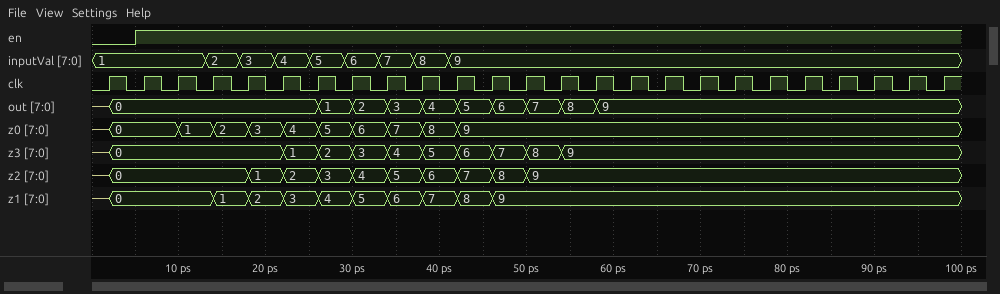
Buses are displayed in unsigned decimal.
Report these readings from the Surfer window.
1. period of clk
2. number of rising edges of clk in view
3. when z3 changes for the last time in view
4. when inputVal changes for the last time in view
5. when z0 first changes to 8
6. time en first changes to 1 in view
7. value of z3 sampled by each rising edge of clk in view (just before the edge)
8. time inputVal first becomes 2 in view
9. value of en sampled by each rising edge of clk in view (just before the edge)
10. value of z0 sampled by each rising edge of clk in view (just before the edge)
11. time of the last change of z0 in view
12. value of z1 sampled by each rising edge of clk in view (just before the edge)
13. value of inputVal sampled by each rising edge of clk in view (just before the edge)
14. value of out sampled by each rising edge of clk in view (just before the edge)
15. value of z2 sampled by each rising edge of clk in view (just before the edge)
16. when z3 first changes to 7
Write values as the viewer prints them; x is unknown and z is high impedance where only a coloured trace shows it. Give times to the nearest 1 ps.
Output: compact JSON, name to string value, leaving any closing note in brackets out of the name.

{"period of clk": "4 ps", "number of rising edges of clk in view": "25", "when z3 changes for the last time in view": "54 ps", "when inputVal changes for the last time in view": "41 ps", "when z0 first changes to 8": "38 ps", "time en first changes to 1 in view": "5 ps", "value of z3 sampled by each rising edge of clk in view": "z, 0, 0, 0, 0, 0, 1, 2, 3, 4, 5, 6, 7, 8, 9, 9, 9, 9, 9, 9, 9, 9, 9, 9, 9", "time inputVal first becomes 2 in view": "13 ps", "value of en sampled by each rising edge of clk in view": "0 1 1 1 1 1 1 1 1 1 1 1 1 1 1 1 1 1 1 1 1 1 1 1 1", "value of z0 sampled by each rising edge of clk in view": "z, 0, 0, 1, 2, 3, 4, 5, 6, 7, 8, 9, 9, 9, 9, 9, 9, 9, 9, 9, 9, 9, 9, 9, 9", "time of the last change of z0 in view": "42 ps", "value of z1 sampled by each rising edge of clk in view": "z, 0, 0, 0, 1, 2, 3, 4, 5, 6, 7, 8, 9, 9, 9, 9, 9, 9, 9, 9, 9, 9, 9, 9, 9", "value of inputVal sampled by each rising edge of clk in view": "1, 1, 1, 2, 3, 4, 5, 6, 7, 8, 9, 9, 9, 9, 9, 9, 9, 9, 9, 9, 9, 9, 9, 9, 9", "value of out sampled by each rising edge of clk in view": "z, 0, 0, 0, 0, 0, 0, 1, 2, 3, 4, 5, 6, 7, 8, 9, 9, 9, 9, 9, 9, 9, 9, 9, 9", "value of z2 sampled by each rising edge of clk in view": "z, 0, 0, 0, 0, 1, 2, 3, 4, 5, 6, 7, 8, 9, 9, 9, 9, 9, 9, 9, 9, 9, 9, 9, 9", "when z3 first changes to 7": "46 ps"}
